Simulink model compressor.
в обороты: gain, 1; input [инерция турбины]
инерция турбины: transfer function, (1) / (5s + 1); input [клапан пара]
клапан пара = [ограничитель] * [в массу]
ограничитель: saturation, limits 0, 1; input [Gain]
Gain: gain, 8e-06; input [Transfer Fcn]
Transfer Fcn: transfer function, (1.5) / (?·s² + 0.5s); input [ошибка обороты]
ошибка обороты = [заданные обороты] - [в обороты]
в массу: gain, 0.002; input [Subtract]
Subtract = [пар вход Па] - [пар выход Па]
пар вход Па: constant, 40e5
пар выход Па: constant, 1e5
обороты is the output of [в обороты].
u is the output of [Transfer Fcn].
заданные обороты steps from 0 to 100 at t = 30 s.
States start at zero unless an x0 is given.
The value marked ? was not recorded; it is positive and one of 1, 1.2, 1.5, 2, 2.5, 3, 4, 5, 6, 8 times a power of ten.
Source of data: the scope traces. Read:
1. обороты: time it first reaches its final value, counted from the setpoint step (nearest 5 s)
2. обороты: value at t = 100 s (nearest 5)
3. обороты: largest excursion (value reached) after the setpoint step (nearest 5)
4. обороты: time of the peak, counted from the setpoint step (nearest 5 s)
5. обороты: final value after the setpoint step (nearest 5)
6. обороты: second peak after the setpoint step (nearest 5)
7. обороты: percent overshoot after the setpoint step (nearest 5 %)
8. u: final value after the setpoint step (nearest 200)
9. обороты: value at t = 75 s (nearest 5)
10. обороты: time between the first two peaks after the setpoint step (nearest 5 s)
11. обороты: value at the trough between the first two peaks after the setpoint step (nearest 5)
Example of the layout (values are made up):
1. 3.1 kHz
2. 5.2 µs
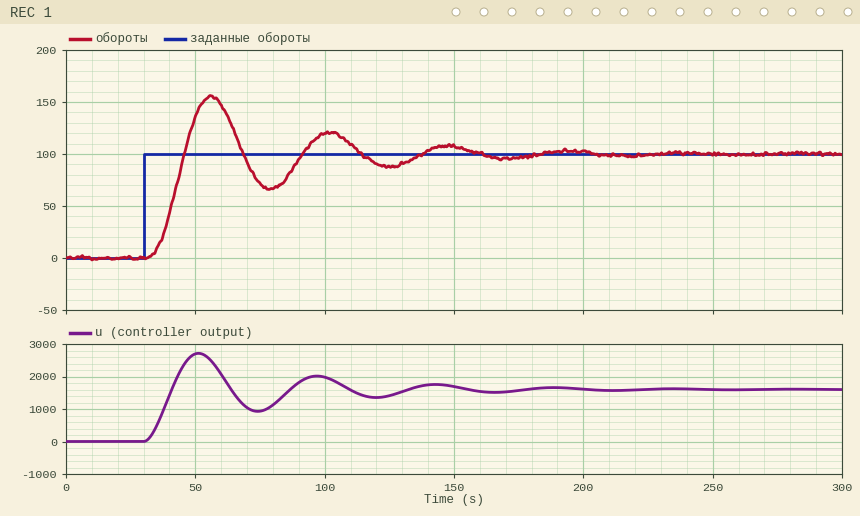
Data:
1. 15 s
2. 120
3. 155
4. 25 s
5. 100
6. 120
7. 55 %
8. 1600
9. 70
10. 45 s
11. 65
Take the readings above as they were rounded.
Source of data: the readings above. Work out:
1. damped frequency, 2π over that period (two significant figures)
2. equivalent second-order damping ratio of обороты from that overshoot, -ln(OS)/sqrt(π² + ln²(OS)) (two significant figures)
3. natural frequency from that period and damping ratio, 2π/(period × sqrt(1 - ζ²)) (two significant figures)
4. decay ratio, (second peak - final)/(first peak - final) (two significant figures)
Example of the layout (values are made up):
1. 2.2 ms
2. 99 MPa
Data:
1. 0.14 rad/s
2. 0.19
3. 0.14 rad/s
4. 0.36
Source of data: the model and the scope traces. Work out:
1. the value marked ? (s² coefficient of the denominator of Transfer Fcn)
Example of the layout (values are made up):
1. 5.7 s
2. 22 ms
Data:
1. 3
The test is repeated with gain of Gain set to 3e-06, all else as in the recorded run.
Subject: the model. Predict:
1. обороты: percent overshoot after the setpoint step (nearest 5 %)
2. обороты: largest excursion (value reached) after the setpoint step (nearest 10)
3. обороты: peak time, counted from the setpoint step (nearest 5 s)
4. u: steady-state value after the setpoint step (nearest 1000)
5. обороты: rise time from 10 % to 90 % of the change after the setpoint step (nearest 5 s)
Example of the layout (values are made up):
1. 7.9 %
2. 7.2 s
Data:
1. 15 %
2. 120
3. 45 s
4. 4000
5. 20 s
